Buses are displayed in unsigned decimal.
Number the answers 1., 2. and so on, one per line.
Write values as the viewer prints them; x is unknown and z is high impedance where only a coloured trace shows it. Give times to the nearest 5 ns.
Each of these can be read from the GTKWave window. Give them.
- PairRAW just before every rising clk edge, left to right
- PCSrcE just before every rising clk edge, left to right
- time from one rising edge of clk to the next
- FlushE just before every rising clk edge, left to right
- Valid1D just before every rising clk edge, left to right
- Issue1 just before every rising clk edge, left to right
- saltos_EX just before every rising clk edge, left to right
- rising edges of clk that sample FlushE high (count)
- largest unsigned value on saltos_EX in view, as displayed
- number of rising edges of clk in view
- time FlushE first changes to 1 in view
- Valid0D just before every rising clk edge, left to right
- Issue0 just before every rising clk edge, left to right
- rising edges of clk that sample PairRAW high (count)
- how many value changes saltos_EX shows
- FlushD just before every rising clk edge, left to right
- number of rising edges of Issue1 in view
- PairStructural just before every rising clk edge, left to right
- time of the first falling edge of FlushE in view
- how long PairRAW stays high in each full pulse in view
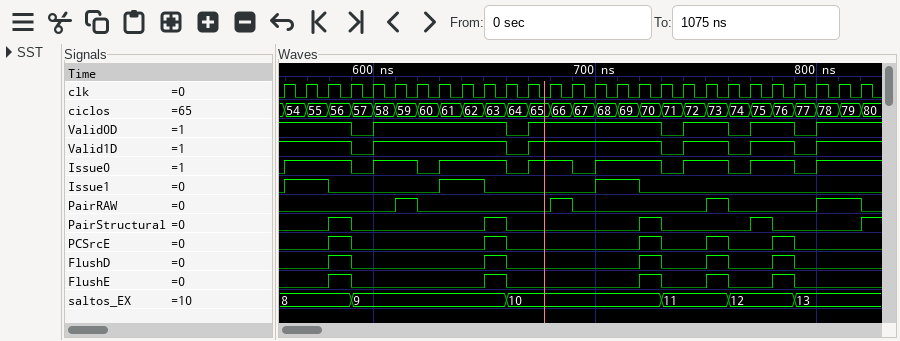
1. 0 0 0 0 0 0 1 0 0 0 0 0 0 1 0 0 0 0 0 0 1 0 0 0 0 1 1
2. 0 0 0 1 0 0 0 0 0 0 1 0 0 0 0 0 0 1 0 0 1 0 0 1 0 0 0
3. 10 ns
4. 0 0 0 1 0 0 0 0 0 0 1 0 0 0 0 0 0 1 0 0 1 0 0 1 0 0 0
5. 1 1 1 1 0 1 1 1 1 1 1 0 1 1 1 1 1 1 0 1 1 0 1 1 0 1 1
6. 0 1 1 0 0 0 0 0 1 1 0 0 0 0 0 1 1 0 0 0 0 0 0 0 0 0 0
7. 8, 8, 8, 8, 9, 9, 9, 9, 9, 9, 9, 10, 10, 10, 10, 10, 10, 10, 11, 11, 11, 12, 12, 12, 13, 13, 13
8. 5
9. 13
10. 27
11. 580 ns
12. 1 1 1 1 0 1 1 1 1 1 1 0 1 1 1 1 1 1 0 1 1 0 1 1 0 1 1
13. 0 1 1 1 0 1 1 0 1 1 1 0 1 1 0 1 1 1 0 1 1 0 1 1 0 1 1
14. 5
15. 5
16. 0 0 0 1 0 0 0 0 0 0 1 0 0 0 0 0 0 1 0 0 1 0 0 1 0 0 0
17. 3
18. 0 0 0 1 0 0 0 0 0 0 1 0 0 0 0 0 0 1 0 0 0 0 1 0 0 0 0
19. 590 ns
20. 10 ns, 10 ns, 10 ns, 20 ns
